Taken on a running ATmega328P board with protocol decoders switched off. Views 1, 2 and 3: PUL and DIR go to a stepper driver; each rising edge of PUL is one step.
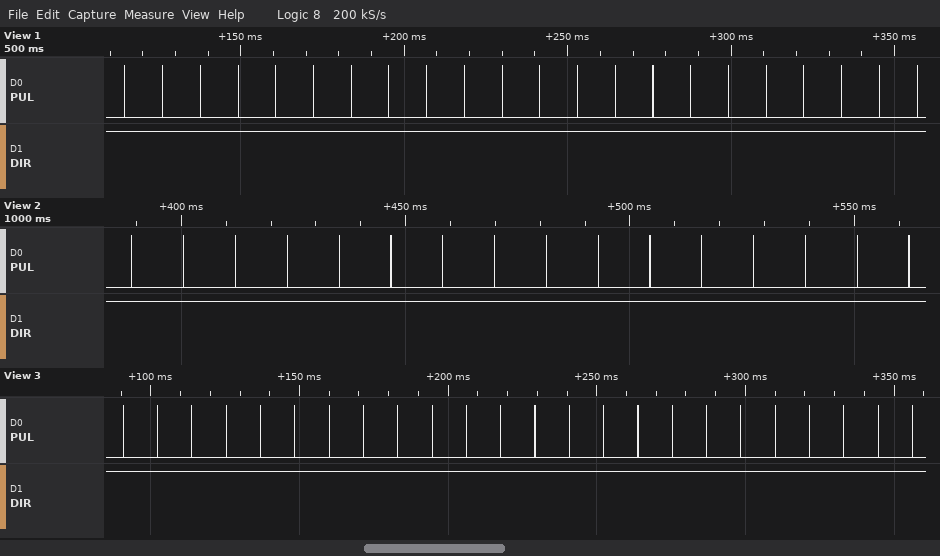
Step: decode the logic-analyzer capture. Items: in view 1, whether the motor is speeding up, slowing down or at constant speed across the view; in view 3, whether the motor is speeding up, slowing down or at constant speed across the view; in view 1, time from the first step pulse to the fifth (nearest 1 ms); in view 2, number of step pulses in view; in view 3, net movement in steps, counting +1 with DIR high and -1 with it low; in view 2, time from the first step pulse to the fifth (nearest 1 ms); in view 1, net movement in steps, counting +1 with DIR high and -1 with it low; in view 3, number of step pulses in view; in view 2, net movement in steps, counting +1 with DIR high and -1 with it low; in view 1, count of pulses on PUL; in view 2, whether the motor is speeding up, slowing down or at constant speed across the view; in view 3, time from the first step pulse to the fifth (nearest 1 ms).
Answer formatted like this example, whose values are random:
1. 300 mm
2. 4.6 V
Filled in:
1. constant speed
2. constant speed
3. 46 ms
4. 16
5. +24
6. 46 ms
7. +22
8. 24
9. +16
10. 22
11. constant speed
12. 46 ms
